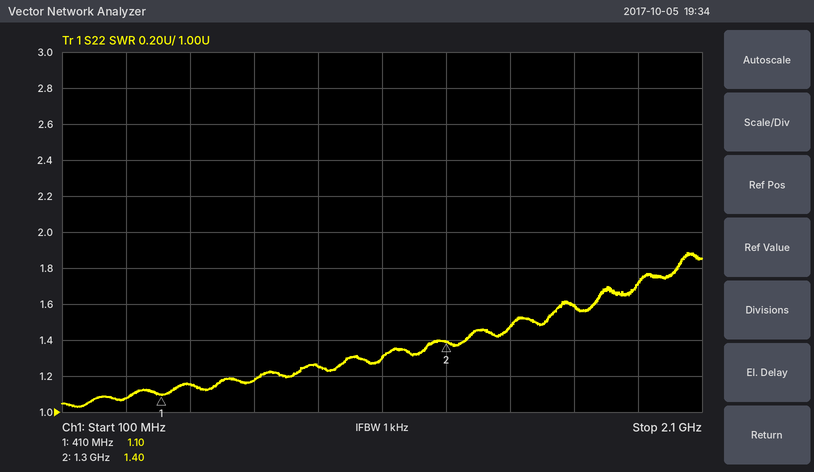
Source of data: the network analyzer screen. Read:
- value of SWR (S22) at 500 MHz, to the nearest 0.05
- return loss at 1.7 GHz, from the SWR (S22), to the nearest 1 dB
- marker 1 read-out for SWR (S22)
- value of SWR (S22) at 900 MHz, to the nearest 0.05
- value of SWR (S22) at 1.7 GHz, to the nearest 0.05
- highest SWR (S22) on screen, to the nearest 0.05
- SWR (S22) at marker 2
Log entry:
1.15
13 dB
1.10
1.25
1.60
1.90
1.40
